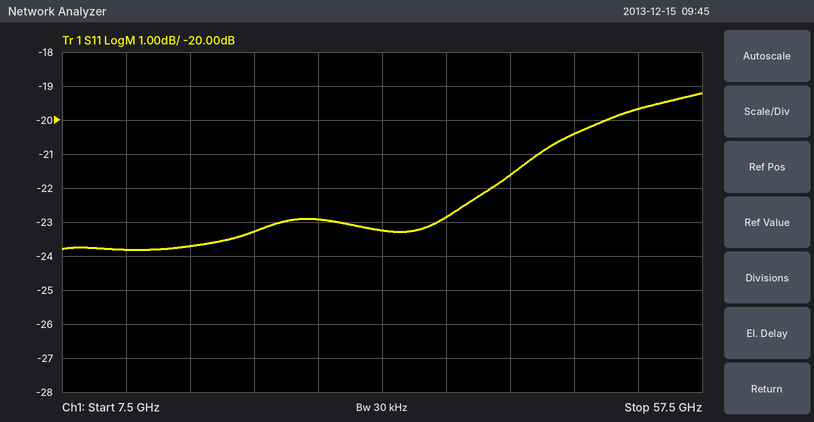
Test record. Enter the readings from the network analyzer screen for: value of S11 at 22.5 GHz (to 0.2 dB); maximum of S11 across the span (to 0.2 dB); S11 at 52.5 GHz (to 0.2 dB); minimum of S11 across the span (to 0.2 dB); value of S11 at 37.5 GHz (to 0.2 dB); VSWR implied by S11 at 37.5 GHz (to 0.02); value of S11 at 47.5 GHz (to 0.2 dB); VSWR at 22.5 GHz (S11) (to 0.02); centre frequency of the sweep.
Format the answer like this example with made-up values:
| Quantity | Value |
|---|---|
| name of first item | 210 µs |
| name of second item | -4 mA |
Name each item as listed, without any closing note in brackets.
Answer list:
| Quantity | Value |
|---|---|
| value of S11 at 22.5 GHz | -23.2 dB |
| maximum of S11 across the span | -19.2 dB |
| S11 at 52.5 GHz | -19.6 dB |
| minimum of S11 across the span | -23.8 dB |
| value of S11 at 37.5 GHz | -22.8 dB |
| VSWR implied by S11 at 37.5 GHz | 1.16 |
| value of S11 at 47.5 GHz | -20.4 dB |
| VSWR at 22.5 GHz (S11) | 1.14 |
| centre frequency of the sweep | 32.5 GHz |
